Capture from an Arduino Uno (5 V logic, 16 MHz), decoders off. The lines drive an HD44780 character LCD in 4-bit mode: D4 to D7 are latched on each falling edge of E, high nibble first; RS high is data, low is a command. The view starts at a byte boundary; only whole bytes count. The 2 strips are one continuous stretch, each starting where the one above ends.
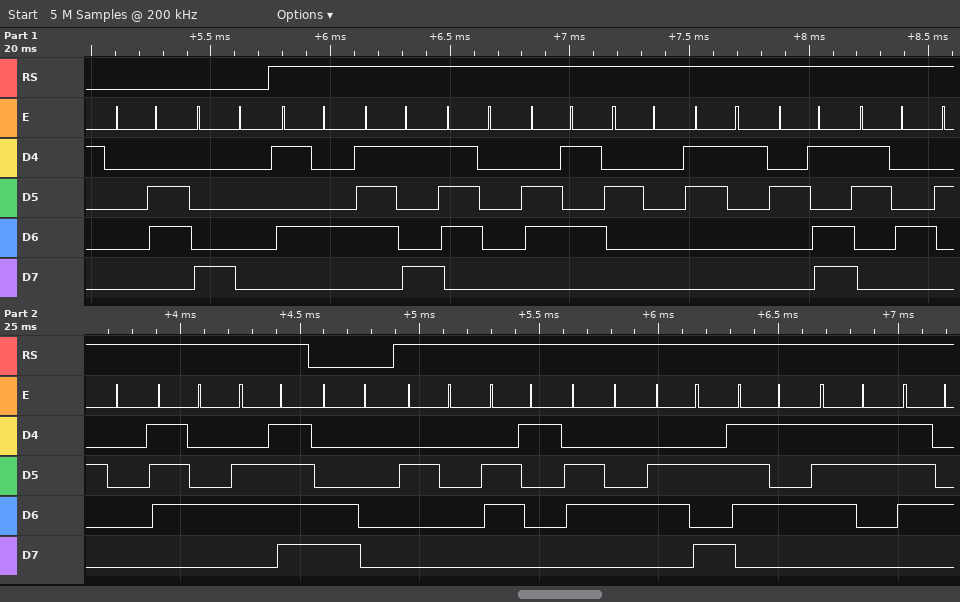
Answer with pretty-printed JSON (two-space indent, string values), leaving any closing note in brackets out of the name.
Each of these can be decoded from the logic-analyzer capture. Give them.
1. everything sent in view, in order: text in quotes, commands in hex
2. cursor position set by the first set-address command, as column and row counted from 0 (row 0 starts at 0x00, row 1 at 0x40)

{
  "everything sent in view, in order: text in quotes, commands in hex": "0x06 0x80 \"Type 1-4 to\" 0xC0 \" adjust\"",
  "cursor position set by the first set-address command, as column and row counted from 0": "column 0, row 0"
}
